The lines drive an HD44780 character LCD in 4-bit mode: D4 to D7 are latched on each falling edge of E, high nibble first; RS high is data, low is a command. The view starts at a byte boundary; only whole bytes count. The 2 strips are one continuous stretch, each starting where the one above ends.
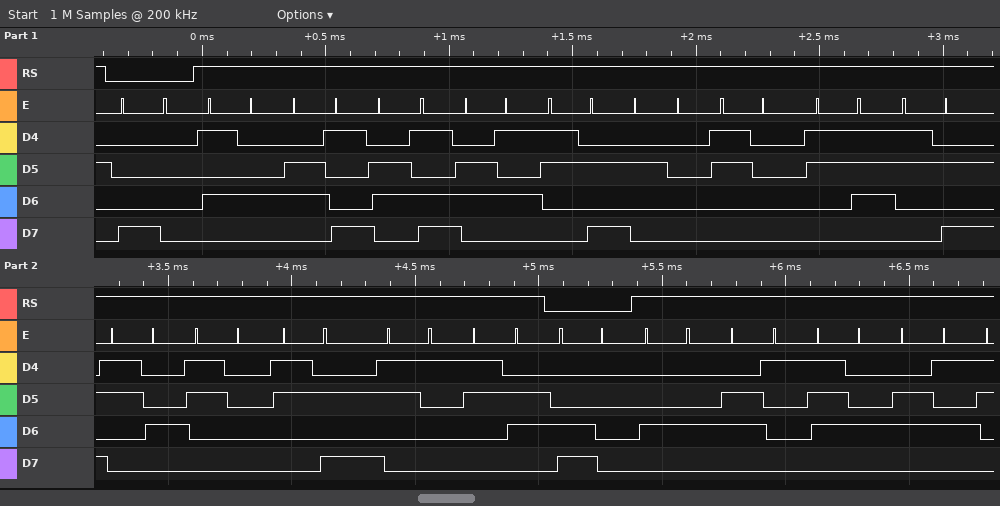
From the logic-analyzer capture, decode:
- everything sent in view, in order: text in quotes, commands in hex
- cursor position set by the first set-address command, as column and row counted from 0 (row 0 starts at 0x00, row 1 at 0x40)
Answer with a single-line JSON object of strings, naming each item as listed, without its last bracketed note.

{"everything sent in view, in order: text in quotes, commands in hex": "0x80 \"Time: 07:40:16\" 0xC0 \"Date\"", "cursor position set by the first set-address command, as column and row counted from 0": "column 0, row 0"}
